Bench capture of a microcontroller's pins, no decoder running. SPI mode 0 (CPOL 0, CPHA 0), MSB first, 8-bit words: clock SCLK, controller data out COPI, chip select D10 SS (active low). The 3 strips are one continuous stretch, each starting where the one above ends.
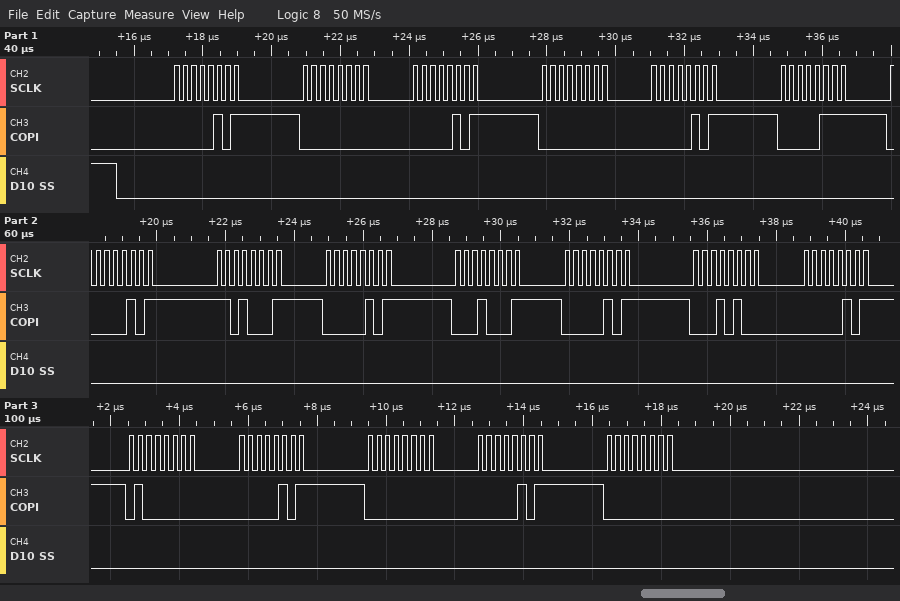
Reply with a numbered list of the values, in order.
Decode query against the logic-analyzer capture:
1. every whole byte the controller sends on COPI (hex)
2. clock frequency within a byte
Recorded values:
1. 05 00 05 00 05 07 05 D1 05 11 05 14 05 40 05 00 05 00
2. 4 MHz
